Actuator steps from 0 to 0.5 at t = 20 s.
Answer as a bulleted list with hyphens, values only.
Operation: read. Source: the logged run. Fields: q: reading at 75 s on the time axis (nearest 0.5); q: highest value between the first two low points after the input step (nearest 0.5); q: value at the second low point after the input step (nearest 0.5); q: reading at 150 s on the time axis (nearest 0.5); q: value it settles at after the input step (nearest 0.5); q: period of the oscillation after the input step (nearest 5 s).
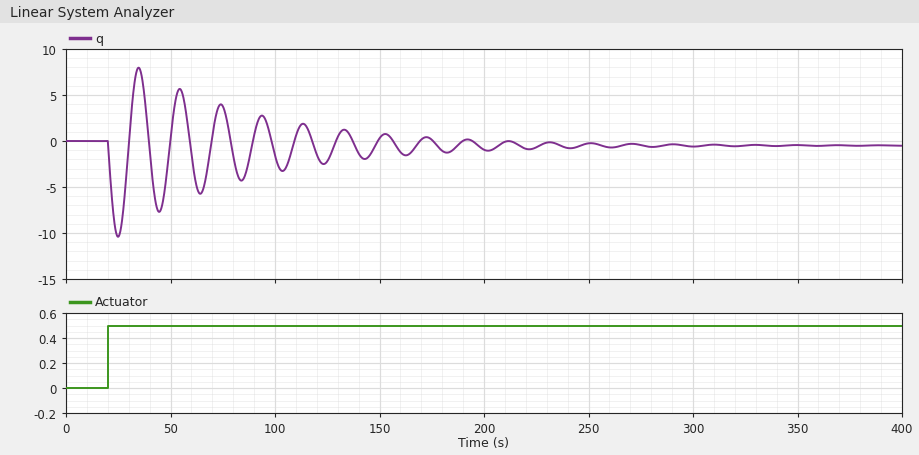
- 4.0
- 8.0
- -7.5
- 0.5
- -0.5
- 20 s
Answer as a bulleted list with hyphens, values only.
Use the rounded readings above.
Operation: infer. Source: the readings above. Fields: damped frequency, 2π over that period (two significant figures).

- 0.31 rad/s
